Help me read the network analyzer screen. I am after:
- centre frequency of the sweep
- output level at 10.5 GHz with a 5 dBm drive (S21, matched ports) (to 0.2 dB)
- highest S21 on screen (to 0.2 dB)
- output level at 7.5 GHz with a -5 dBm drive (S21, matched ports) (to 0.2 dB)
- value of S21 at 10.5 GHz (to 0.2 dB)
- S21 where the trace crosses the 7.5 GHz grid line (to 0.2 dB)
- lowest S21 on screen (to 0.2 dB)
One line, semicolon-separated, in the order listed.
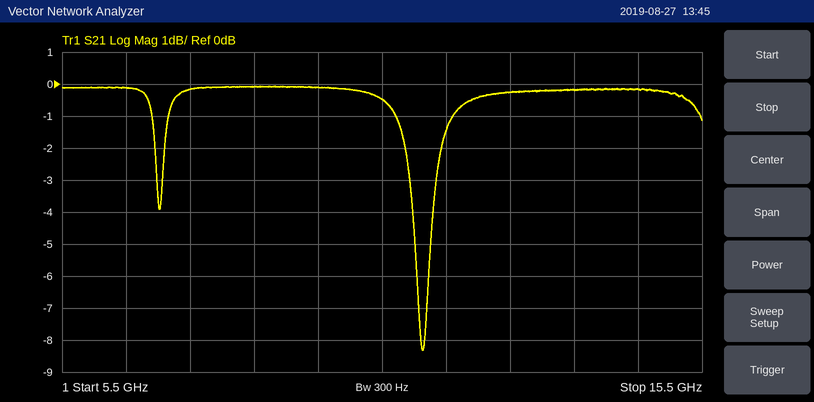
10.5 GHz; 4.6 dBm; 0.0 dB; -5.2 dBm; -0.4 dB; -0.2 dB; -8.4 dB
